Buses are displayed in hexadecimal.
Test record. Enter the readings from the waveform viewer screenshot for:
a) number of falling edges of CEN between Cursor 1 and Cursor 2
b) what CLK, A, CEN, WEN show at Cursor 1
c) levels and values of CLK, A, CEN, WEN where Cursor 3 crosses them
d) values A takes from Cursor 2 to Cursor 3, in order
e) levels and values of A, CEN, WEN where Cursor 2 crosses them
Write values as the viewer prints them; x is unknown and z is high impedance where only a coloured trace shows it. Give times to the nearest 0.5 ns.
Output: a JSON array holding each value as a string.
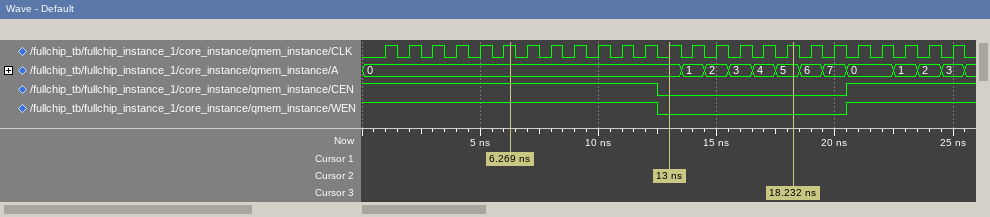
["1", "CLK=1, A=0, CEN=1, WEN=1", "CLK=1, A=5, CEN=0, WEN=0", "0, 1, 2, 3, 4, 5", "A=0, CEN=0, WEN=0"]
